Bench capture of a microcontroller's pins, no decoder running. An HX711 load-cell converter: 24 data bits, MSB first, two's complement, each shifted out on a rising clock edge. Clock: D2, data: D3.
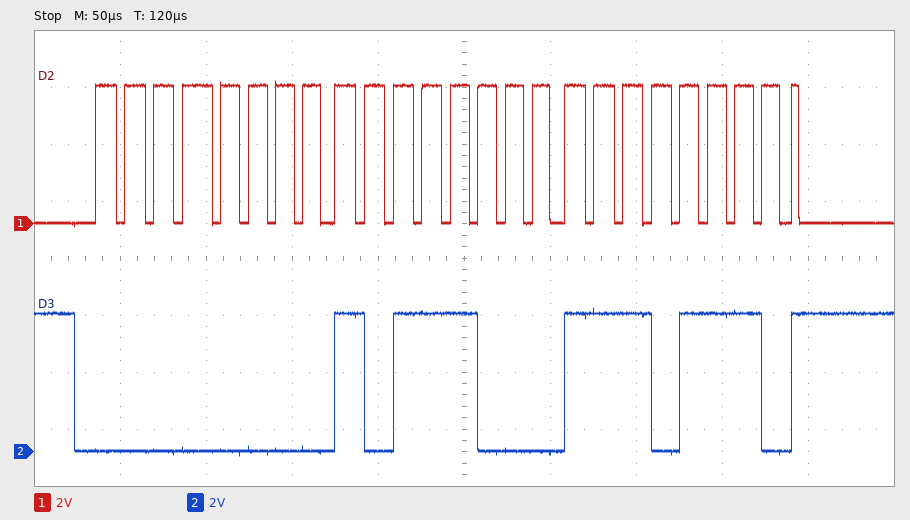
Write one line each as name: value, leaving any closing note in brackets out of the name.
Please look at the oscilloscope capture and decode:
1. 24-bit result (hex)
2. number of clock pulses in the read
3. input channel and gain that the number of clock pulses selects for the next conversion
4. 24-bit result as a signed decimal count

24-bit result: 0x00B8EE
number of clock pulses in the read: 25
input channel and gain that the number of clock pulses selects for the next conversion: channel A, gain 128
24-bit result as a signed decimal count: 47342
